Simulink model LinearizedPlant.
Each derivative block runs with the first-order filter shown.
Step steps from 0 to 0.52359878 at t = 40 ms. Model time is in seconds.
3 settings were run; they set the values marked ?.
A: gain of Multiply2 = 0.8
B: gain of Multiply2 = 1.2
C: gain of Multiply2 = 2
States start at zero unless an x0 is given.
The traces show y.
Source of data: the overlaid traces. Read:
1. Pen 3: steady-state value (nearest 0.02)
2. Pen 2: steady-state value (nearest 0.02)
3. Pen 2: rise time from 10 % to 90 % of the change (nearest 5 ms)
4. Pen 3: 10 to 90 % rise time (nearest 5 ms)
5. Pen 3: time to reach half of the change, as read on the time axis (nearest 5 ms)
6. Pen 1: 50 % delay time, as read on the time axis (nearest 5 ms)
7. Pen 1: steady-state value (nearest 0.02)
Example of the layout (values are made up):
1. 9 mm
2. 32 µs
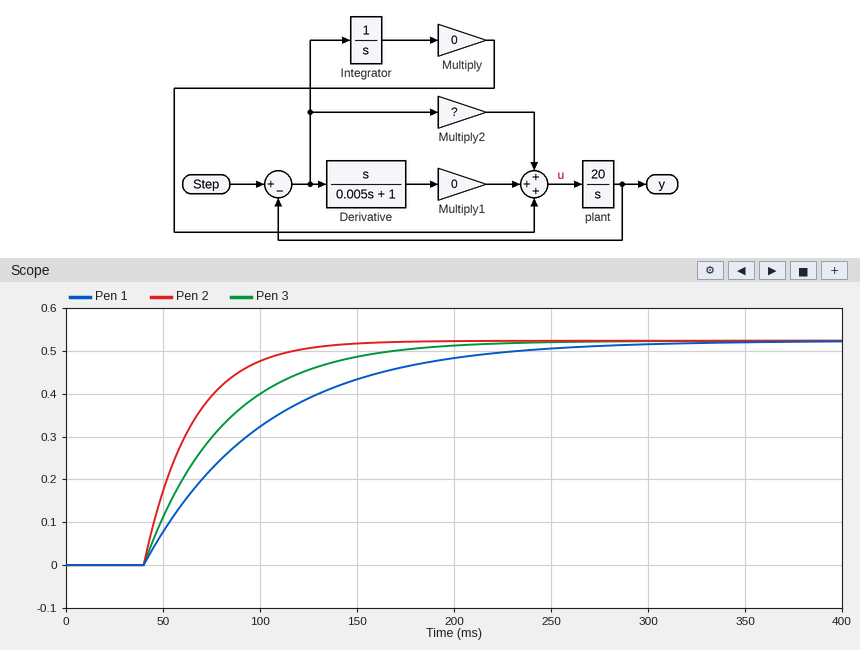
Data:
1. 0.52
2. 0.52
3. 55 ms
4. 90 ms
5. 70 ms
6. 85 ms
7. 0.52
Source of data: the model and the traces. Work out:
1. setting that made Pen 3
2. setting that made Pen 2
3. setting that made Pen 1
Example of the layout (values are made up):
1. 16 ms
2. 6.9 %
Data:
1. B
2. C
3. A
